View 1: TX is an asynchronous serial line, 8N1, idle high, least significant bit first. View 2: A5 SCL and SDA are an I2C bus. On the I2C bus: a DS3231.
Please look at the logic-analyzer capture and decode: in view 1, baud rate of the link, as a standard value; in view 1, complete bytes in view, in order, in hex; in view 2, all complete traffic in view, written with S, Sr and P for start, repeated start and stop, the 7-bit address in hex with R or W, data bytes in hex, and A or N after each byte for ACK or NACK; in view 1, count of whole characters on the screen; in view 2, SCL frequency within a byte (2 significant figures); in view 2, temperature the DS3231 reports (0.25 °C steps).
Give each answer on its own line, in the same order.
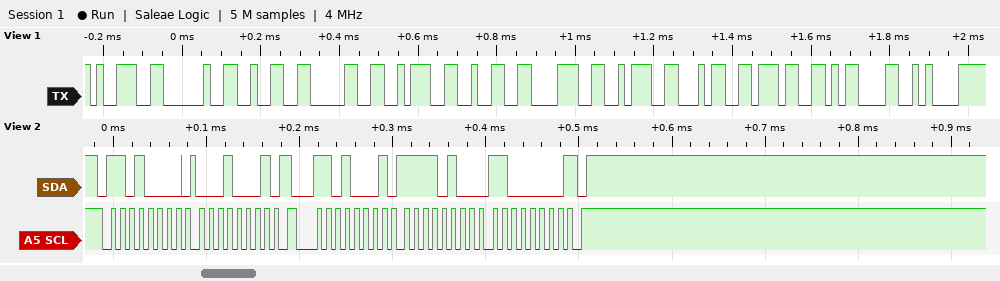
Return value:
57600 baud
39 20 32 30 3A 32 38 3A 34 37 0D 0A
S 68W A 11 A Sr 68R A F4 A C0 N P
12
100 kHz
-11.25 °C
